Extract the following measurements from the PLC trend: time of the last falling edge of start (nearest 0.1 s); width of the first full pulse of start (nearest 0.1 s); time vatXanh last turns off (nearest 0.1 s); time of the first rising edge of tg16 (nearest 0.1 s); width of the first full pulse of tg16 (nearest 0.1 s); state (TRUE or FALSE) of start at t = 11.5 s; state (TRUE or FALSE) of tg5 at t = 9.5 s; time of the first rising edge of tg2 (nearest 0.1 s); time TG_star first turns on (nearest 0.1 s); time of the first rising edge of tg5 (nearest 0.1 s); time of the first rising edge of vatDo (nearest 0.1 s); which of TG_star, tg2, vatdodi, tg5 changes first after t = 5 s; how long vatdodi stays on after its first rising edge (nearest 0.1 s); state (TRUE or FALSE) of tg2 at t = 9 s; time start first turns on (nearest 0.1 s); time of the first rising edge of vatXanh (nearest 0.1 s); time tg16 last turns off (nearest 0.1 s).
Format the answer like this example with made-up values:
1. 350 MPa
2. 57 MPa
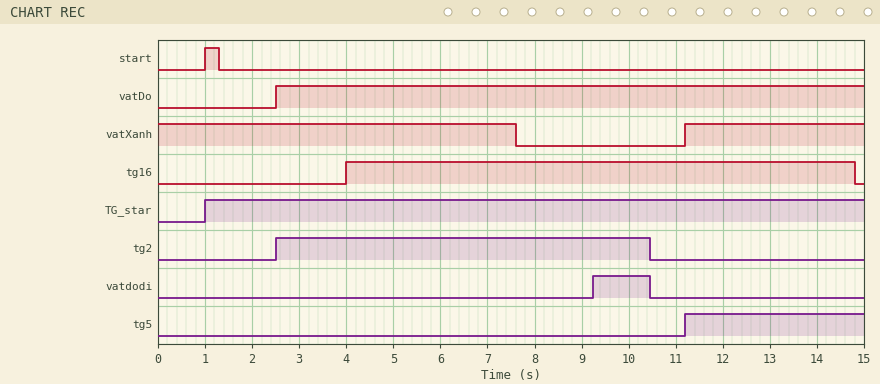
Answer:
1. 1.3 s
2. 0.3 s
3. 7.6 s
4. 4.0 s
5. 10.8 s
6. FALSE
7. FALSE
8. 2.5 s
9. 1.0 s
10. 11.2 s
11. 2.5 s
12. vatdodi
13. 1.2 s
14. TRUE
15. 1.0 s
16. 11.2 s
17. 14.8 s
